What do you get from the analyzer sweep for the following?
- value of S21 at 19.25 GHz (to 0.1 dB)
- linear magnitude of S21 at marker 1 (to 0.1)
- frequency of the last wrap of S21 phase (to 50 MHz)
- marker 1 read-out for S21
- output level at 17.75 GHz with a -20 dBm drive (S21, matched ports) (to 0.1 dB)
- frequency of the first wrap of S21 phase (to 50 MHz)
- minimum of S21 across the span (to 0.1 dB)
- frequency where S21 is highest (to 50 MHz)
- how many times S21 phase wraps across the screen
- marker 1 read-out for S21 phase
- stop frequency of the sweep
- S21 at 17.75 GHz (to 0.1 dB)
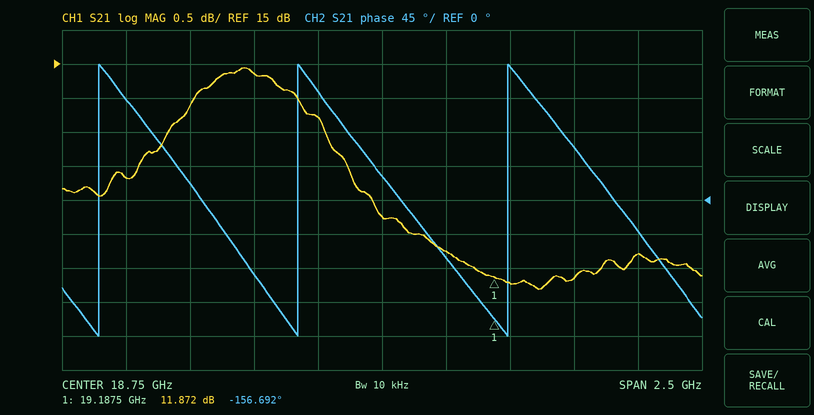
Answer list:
11.8 dB
3.9
19.25 GHz
11.872 dB
-6.7 dBm
17.65 GHz
11.7 dB
18.20 GHz
3
-156.692°
20 GHz
13.3 dB
